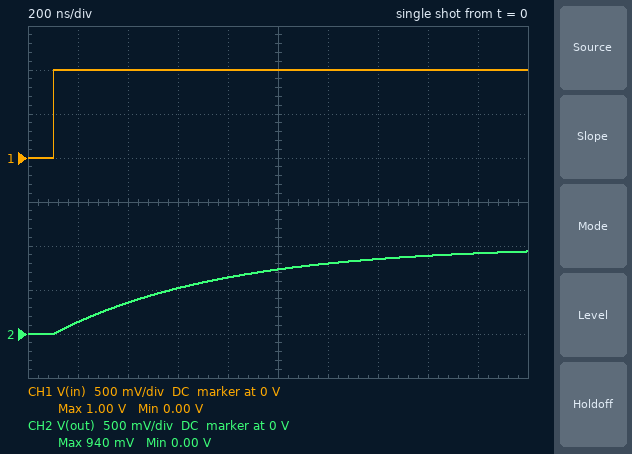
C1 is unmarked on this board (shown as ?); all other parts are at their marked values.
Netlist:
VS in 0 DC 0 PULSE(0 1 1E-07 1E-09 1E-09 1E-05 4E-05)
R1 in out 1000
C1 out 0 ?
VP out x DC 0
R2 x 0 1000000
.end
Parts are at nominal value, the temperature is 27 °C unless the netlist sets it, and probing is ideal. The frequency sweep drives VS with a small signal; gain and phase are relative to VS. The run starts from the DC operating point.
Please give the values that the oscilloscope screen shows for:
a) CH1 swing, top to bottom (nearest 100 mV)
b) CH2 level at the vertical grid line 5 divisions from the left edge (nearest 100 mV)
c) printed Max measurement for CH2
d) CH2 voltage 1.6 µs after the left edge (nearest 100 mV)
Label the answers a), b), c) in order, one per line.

a) 1.0 V
b) 700 mV
c) 940 mV
d) 900 mV
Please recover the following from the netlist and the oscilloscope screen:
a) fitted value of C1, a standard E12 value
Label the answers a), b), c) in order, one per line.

a) 680 pF
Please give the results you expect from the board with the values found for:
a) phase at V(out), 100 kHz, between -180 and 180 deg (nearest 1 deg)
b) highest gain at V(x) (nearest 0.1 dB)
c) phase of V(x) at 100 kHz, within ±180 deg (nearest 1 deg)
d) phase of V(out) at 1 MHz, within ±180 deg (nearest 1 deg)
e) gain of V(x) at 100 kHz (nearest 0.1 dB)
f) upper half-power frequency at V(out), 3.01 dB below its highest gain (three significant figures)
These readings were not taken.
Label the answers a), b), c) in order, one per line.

a) -23 deg
b) 0 dB
c) -23 deg
d) -77 deg
e) -0.7 dB
f) 234 kHz
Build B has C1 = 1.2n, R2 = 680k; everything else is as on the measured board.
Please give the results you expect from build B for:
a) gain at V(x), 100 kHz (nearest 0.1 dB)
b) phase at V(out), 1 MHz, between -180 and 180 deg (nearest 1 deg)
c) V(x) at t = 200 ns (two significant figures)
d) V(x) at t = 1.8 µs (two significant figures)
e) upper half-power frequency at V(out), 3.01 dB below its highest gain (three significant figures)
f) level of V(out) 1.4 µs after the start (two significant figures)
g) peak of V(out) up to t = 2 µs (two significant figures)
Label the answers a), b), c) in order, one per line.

a) -2.0 dB
b) -82 deg
c) 80 mV
d) 760 mV
e) 133 kHz
f) 660 mV
g) 790 mV
